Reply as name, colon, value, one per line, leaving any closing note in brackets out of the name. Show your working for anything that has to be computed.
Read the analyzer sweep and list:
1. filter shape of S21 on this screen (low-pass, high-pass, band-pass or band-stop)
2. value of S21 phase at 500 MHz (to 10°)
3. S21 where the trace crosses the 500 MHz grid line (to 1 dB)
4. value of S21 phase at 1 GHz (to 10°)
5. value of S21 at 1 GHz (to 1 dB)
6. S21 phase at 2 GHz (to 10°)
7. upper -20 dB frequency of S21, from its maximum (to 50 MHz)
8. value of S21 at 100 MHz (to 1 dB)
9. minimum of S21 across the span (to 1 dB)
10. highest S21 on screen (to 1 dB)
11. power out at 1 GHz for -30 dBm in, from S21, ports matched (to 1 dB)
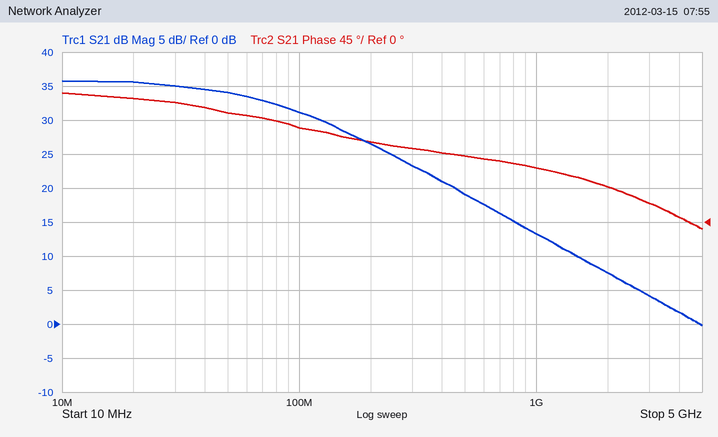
filter shape of S21 on this screen: low-pass
value of S21 phase at 500 MHz: 90°
S21 where the trace crosses the 500 MHz grid line: 19 dB
value of S21 phase at 1 GHz: 70°
value of S21 at 1 GHz: 13 dB
S21 phase at 2 GHz: 50°
upper -20 dB frequency of S21, from its maximum: 750 MHz
value of S21 at 100 MHz: 31 dB
minimum of S21 across the span: 0 dB
highest S21 on screen: 36 dB
power out at 1 GHz for -30 dBm in, from S21, ports matched: -30 dBm + (13 dB) = -17 dBm
